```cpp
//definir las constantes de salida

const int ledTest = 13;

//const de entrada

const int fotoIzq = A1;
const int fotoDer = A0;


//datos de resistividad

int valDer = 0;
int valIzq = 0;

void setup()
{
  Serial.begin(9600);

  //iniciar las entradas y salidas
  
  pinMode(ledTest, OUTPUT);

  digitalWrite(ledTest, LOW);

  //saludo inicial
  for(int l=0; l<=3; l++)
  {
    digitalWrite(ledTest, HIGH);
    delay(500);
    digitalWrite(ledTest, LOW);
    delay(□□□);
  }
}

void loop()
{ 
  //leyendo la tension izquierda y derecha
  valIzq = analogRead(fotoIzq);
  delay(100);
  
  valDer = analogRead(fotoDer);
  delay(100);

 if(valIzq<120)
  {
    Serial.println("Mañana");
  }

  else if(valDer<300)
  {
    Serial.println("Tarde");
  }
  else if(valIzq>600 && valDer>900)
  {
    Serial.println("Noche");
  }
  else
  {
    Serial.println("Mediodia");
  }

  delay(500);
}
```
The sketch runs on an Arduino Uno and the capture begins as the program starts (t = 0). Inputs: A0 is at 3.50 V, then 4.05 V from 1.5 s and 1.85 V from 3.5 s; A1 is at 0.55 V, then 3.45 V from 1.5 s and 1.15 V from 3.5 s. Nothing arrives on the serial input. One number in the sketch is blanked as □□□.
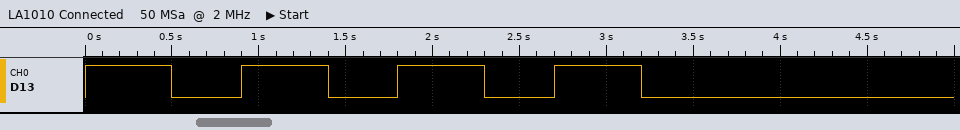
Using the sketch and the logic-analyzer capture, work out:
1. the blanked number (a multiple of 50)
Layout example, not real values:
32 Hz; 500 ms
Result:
400
